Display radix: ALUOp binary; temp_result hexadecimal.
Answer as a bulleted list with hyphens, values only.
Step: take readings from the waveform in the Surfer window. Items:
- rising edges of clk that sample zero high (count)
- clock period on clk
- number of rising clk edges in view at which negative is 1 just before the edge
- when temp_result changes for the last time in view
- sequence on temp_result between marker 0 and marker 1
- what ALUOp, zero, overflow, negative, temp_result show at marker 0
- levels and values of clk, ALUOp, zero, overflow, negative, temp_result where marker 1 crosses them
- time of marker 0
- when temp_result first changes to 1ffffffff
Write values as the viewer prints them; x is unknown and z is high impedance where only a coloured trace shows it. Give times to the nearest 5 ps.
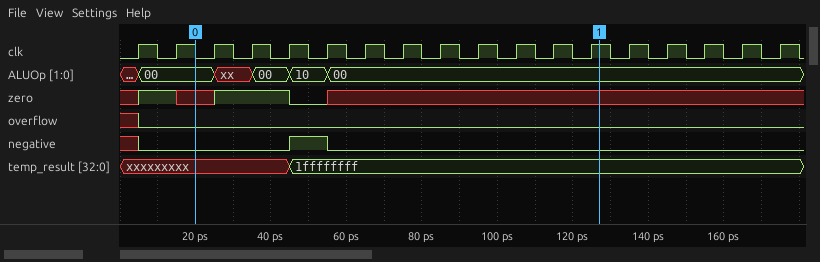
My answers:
- 3
- 10 ps
- 1
- 45 ps
- xxxxxxxxx, 1ffffffff
- ALUOp=00, zero=x, overflow=0, negative=0, temp_result=xxxxxxxxx
- clk=1, ALUOp=00, zero=x, overflow=0, negative=0, temp_result=1ffffffff
- 20 ps
- 45 ps
